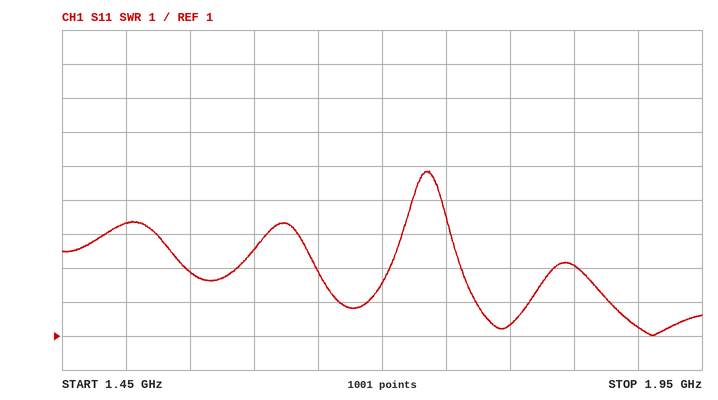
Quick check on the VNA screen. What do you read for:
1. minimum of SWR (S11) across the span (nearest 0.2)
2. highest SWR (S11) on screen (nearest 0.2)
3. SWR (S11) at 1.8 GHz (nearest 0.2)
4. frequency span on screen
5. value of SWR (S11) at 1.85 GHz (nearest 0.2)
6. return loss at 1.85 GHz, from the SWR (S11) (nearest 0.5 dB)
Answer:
1.0
5.8
1.4
500 MHz
3.0
6.0 dB
